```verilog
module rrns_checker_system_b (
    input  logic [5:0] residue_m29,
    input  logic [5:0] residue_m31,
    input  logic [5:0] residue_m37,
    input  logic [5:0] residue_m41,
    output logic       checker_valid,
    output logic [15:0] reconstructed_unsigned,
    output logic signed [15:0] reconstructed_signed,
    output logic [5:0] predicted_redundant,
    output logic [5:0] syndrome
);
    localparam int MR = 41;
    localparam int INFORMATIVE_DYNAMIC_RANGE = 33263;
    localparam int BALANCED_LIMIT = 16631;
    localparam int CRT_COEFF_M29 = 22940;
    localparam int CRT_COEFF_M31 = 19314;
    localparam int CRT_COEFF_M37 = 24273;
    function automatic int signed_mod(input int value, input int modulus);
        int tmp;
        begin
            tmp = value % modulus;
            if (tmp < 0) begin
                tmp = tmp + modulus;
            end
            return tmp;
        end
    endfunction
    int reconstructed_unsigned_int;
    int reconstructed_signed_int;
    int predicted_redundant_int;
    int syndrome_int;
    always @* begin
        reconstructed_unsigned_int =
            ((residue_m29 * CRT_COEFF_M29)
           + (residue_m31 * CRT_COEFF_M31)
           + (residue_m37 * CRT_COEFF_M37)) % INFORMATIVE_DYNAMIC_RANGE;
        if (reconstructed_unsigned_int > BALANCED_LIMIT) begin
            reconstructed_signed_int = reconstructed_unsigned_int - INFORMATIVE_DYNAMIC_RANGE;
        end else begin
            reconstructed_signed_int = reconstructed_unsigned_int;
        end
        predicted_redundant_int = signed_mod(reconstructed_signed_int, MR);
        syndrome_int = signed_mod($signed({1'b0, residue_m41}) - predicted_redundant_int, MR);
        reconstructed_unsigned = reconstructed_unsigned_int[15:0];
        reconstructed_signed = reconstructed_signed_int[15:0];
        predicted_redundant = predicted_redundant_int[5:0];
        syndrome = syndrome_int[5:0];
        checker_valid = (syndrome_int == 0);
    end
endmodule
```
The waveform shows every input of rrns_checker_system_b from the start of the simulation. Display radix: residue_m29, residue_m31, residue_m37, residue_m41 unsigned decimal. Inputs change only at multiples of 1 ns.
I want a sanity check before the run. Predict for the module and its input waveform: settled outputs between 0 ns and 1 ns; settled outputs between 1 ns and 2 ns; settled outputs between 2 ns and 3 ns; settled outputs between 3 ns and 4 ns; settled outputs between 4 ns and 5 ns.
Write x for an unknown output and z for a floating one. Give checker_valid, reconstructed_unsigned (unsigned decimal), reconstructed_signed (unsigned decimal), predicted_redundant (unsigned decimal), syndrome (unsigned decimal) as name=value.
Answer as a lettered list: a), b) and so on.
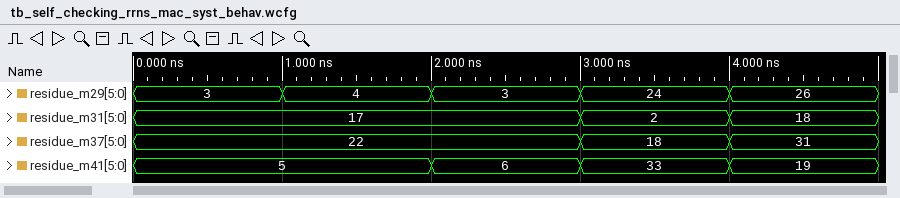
a) checker_valid=1, reconstructed_unsigned=33063, reconstructed_signed=65336, predicted_redundant=5, syndrome=0
b) checker_valid=0, reconstructed_unsigned=22740, reconstructed_signed=55013, predicted_redundant=14, syndrome=32
c) checker_valid=0, reconstructed_unsigned=33063, reconstructed_signed=65336, predicted_redundant=5, syndrome=1
d) checker_valid=1, reconstructed_unsigned=28212, reconstructed_signed=60485, predicted_redundant=33, syndrome=0
e) checker_valid=1, reconstructed_unsigned=142, reconstructed_signed=142, predicted_redundant=19, syndrome=0
